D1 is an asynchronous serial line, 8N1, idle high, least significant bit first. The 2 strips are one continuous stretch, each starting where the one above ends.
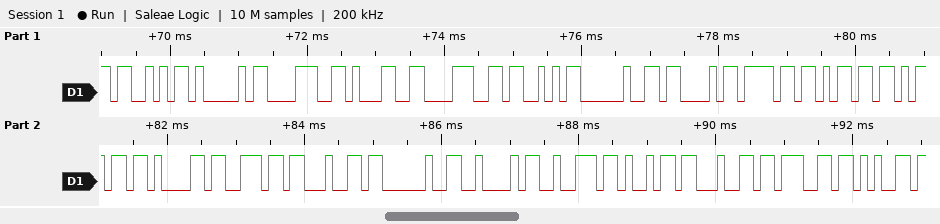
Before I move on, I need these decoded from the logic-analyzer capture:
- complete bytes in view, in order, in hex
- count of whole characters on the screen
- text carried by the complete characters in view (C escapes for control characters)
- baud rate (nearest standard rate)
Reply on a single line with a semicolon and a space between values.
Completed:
53 41 38 31 38 53 20 43 6F 6D 6D 61 6E 64 20 42 72 69 64 67 65; 21; "SA818S Command Bridge"; 9600 baud
